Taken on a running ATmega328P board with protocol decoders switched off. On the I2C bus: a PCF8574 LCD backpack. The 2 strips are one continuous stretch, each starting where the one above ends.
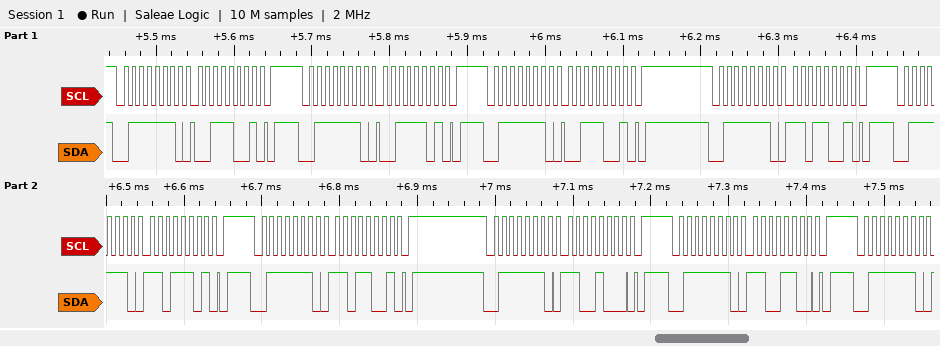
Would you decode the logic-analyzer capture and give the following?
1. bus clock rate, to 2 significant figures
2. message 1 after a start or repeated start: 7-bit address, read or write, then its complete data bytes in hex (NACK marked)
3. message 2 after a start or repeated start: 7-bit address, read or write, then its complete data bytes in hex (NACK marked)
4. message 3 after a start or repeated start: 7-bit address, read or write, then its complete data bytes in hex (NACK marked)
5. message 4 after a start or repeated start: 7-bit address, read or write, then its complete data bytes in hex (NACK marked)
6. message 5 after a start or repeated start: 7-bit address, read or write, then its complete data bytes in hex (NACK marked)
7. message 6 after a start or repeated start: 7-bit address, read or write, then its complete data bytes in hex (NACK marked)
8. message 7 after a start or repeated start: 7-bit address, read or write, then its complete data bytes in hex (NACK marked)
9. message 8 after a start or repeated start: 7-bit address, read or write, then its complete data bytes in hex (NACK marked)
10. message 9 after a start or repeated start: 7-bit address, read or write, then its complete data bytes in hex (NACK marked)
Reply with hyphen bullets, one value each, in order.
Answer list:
- 100 kHz
- 0x3F write: 39
- 0x3F write: 3D
- 0x3F write: 39
- 0x3F write: D9
- 0x3F write: DD
- 0x3F write: D9
- 0x3F write: C8
- 0x3F write: CC
- 0x3F write
